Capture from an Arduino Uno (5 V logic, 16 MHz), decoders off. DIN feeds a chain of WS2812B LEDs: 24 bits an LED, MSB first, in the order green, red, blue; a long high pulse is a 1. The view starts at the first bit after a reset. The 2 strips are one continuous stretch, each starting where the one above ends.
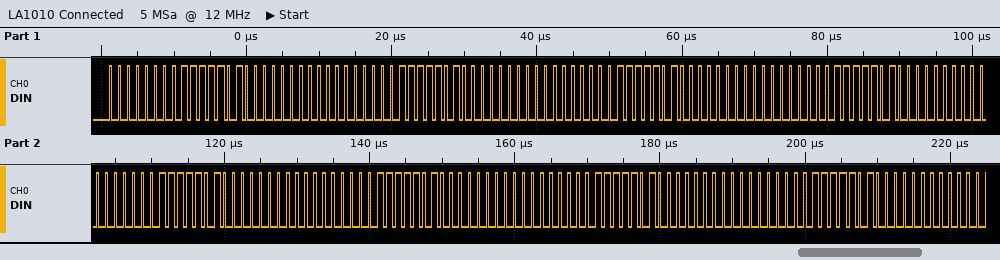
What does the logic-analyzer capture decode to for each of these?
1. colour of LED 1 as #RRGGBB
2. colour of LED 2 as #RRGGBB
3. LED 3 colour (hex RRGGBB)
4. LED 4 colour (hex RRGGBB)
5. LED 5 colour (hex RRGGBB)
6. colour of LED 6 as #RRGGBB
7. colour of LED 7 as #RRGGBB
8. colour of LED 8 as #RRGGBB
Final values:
#FA0000
#FA0000
#FA0000
#FA0000
#FA0000
#FA0000
#FA0000
#FA0000
